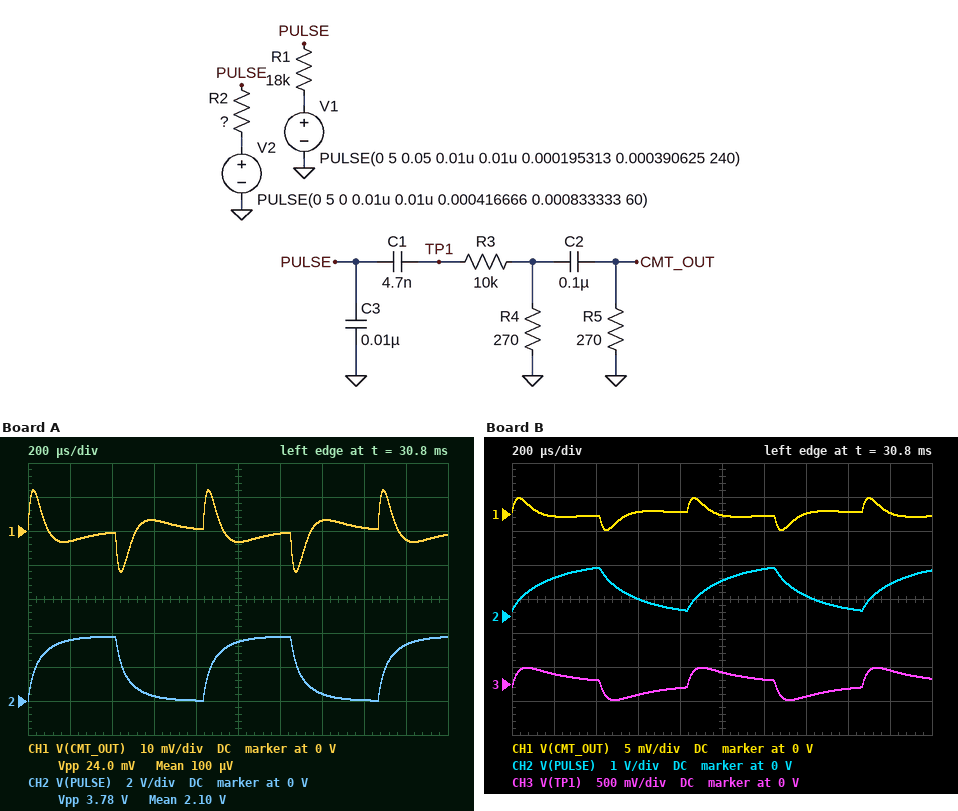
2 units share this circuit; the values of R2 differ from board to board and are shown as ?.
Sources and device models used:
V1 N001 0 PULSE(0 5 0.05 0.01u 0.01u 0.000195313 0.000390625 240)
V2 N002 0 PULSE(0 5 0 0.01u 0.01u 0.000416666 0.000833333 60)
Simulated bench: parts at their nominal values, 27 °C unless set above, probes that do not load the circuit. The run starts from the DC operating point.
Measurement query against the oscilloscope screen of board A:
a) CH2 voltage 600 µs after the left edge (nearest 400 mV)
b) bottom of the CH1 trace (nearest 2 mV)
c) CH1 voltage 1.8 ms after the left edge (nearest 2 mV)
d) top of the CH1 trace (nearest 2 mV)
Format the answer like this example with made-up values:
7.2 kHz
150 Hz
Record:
400 mV
-12 mV
-2 mV
12 mV
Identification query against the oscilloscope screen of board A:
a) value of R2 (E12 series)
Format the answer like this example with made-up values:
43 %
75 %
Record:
5.6 kΩ
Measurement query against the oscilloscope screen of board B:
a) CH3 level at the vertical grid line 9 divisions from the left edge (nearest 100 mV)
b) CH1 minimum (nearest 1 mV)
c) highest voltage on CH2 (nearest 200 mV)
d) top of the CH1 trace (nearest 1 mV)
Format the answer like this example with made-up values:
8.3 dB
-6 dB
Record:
200 mV
-2 mV
1.4 V
2 mV
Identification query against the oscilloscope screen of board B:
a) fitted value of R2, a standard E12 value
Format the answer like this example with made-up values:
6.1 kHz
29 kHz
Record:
39 kΩ
